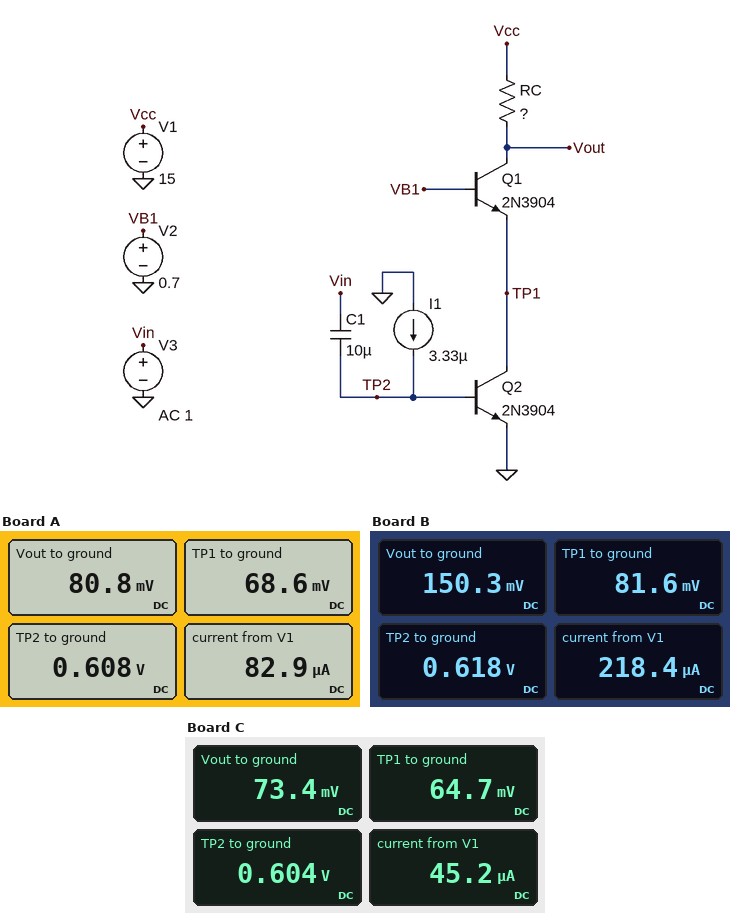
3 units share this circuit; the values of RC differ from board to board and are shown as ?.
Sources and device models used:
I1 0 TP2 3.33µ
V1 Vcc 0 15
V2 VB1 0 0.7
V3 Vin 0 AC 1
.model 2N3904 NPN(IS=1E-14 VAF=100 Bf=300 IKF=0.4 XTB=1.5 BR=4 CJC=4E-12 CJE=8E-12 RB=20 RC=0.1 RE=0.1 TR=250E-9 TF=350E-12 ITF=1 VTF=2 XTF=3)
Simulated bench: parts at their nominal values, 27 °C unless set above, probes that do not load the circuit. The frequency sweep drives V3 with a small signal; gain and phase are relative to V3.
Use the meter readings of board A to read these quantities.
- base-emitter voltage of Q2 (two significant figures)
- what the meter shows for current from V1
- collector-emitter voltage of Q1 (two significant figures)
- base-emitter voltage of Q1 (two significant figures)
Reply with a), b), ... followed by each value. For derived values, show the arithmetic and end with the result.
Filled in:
a) 608 mV = 610 mV
b) 82.9 µA
c) 80.8 mV - 68.6 mV = 12 mV
d) 700 mV - 68.6 mV = 630 mV
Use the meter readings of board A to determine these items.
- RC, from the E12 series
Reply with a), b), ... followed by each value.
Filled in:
a) 180 kΩ
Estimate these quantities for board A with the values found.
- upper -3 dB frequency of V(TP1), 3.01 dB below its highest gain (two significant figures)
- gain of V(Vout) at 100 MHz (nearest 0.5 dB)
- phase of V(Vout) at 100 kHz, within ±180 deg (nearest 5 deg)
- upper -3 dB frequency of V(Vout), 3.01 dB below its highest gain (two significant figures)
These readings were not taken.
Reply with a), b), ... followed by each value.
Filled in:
a) 190 kHz
b) -14.5 dB
c) 150 deg
d) 180 kHz
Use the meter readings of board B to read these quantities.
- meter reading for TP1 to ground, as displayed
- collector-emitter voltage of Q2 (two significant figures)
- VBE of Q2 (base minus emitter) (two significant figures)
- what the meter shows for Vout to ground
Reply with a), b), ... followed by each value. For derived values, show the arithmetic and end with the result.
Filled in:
a) 81.6 mV
b) 81.6 mV = 82 mV
c) 618 mV = 620 mV
d) 150.3 mV
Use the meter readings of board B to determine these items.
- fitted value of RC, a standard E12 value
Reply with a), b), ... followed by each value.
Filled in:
a) 68 kΩ
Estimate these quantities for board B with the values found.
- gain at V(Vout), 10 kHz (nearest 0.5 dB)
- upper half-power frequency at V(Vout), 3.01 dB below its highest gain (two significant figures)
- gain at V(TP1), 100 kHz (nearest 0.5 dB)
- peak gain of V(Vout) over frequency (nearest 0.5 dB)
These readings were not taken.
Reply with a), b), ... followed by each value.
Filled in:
a) 31.5 dB
b) 190 kHz
c) 10.0 dB
d) 31.5 dB
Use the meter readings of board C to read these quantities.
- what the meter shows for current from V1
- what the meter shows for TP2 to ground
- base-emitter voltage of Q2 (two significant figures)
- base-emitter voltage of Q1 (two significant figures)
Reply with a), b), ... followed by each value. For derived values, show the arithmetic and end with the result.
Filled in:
a) 45.2 µA
b) 0.604 V
c) 604 mV = 600 mV
d) 700 mV - 64.7 mV = 640 mV
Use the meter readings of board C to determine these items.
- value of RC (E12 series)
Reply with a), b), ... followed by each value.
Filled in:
a) 330 kΩ
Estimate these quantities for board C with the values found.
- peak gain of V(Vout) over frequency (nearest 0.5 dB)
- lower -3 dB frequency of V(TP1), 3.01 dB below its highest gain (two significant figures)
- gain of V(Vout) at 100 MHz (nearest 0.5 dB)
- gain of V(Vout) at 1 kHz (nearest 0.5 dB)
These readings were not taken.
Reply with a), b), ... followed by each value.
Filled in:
a) 3.0 dB
b) 4.3 Hz
c) -14.0 dB
d) 3.0 dB
